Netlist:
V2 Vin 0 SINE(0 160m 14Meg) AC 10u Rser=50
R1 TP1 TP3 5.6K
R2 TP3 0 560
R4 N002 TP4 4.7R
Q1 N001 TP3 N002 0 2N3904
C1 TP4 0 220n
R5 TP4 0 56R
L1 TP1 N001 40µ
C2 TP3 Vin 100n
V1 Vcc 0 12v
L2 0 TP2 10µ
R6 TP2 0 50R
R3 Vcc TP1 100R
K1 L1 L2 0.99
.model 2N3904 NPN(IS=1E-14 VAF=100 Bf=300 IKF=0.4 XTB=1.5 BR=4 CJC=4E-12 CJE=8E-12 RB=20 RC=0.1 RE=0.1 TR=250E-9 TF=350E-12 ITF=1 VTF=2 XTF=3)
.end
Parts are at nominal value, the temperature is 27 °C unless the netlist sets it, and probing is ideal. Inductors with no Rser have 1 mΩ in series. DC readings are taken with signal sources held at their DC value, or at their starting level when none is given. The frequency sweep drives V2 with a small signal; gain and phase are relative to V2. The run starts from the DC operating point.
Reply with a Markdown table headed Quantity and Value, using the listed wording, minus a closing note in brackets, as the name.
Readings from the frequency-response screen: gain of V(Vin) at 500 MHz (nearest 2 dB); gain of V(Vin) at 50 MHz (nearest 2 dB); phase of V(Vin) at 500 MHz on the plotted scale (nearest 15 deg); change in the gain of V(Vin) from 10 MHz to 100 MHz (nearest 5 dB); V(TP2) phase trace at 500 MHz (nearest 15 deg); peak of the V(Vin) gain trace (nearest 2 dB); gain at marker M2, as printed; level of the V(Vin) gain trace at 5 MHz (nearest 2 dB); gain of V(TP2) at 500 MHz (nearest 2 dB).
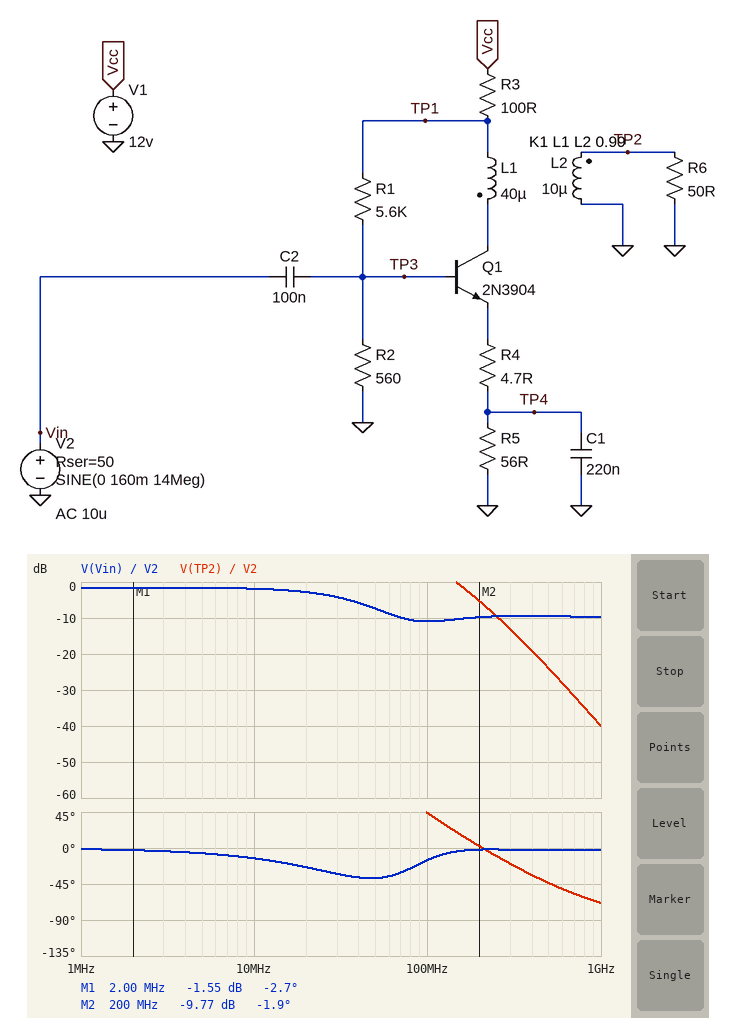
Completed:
| Quantity | Value |
|---|---|
| gain of V(Vin) at 500 MHz | -10 dB |
| gain of V(Vin) at 50 MHz | -8 dB |
| phase of V(Vin) at 500 MHz on the plotted scale | 0 deg |
| change in the gain of V(Vin) from 10 MHz to 100 MHz | -10 dB |
| V(TP2) phase trace at 500 MHz | -45 deg |
| peak of the V(Vin) gain trace | -2 dB |
| gain at marker M2, as printed | -9.77 dB |
| level of the V(Vin) gain trace at 5 MHz | -2 dB |
| gain of V(TP2) at 500 MHz | -24 dB |
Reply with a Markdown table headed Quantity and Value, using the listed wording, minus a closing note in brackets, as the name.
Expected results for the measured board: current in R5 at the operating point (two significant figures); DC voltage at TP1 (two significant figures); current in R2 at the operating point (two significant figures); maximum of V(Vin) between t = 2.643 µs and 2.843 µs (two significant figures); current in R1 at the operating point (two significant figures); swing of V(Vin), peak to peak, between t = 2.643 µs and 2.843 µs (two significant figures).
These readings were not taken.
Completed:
| Quantity | Value |
|---|---|
| current in R5 at the operating point | 5.3 mA |
| DC voltage at TP1 | 11 V |
| current in R2 at the operating point | 1.8 mA |
| maximum of V(Vin) between t = 2.643 µs and 2.843 µs | 120 mV |
| current in R1 at the operating point | 1.8 mA |
| swing of V(Vin), peak to peak, between t = 2.643 µs and 2.843 µs | 260 mV |
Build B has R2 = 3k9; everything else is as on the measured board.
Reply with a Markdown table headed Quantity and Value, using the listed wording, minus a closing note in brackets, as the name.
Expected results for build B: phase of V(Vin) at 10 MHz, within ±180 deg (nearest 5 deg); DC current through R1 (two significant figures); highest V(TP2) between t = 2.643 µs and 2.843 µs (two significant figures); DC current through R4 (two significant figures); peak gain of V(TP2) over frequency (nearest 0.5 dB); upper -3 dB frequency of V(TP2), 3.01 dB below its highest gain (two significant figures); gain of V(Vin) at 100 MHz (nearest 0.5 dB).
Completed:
| Quantity | Value |
|---|---|
| phase of V(Vin) at 10 MHz, within ±180 deg | -20 deg |
| DC current through R1 | 910 µA |
| highest V(TP2) between t = 2.643 µs and 2.843 µs | 1.9 V |
| DC current through R4 | 38 mA |
| peak gain of V(TP2) over frequency | 23.0 dB |
| upper -3 dB frequency of V(TP2), 3.01 dB below its highest gain | 19 MHz |
| gain of V(Vin) at 100 MHz | -10.5 dB |
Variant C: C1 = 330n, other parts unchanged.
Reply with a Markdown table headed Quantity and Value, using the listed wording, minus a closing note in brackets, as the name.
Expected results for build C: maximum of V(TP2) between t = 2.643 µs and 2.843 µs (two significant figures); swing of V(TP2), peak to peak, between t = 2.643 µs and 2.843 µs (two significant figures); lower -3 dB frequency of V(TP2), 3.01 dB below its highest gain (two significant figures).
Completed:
| Quantity | Value |
|---|---|
| maximum of V(TP2) between t = 2.643 µs and 2.843 µs | 780 mV |
| swing of V(TP2), peak to peak, between t = 2.643 µs and 2.843 µs | 1.9 V |
| lower -3 dB frequency of V(TP2), 3.01 dB below its highest gain | 770 kHz |
